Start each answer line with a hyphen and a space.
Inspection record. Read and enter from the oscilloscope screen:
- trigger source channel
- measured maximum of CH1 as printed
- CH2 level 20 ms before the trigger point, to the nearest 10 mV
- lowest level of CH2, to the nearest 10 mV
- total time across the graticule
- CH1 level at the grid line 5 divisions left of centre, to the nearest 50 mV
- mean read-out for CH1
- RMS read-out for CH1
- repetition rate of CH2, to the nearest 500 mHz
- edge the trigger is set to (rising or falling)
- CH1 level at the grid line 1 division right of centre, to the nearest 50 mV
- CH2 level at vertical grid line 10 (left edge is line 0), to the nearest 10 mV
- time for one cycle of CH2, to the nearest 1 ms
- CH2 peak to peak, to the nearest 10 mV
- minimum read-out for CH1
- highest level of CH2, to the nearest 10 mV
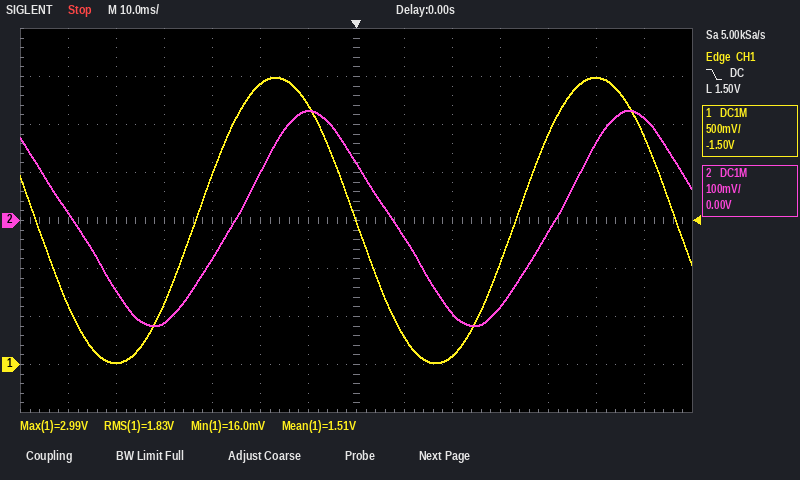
- CH1
- 2.99 V
- 100 mV
- -220 mV
- 140 ms
- 0 mV
- 1.51 V
- 1.83 V
- 15.0 Hz
- falling
- 300 mV
- -180 mV
- 67 ms
- 450 mV
- 16.0 mV
- 230 mV
